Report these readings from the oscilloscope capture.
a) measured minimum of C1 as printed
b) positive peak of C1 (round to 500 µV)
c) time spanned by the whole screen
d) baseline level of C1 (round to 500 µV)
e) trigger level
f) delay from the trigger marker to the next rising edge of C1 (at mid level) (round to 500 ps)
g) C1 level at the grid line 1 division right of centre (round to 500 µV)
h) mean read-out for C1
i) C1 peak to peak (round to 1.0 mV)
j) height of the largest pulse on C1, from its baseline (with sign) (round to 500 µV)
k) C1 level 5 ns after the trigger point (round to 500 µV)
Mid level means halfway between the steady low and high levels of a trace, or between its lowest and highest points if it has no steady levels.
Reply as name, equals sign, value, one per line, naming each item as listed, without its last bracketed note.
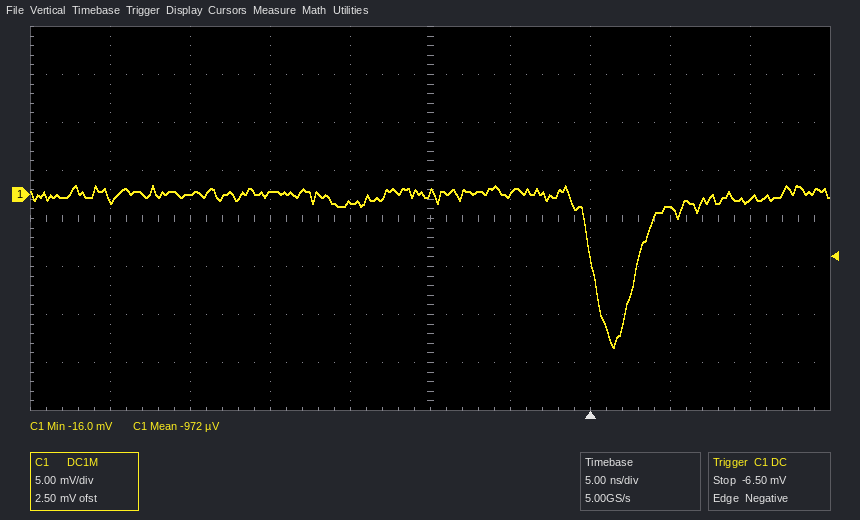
measured minimum of C1 as printed = -16.0 mV
positive peak of C1 = 1.0 mV
time spanned by the whole screen = 50 ns
baseline level of C1 = 0.0 mV
trigger level = -6.50 mV
delay from the trigger marker to the next rising edge of C1 (at mid level) = 3.0 ns
C1 level at the grid line 1 division right of centre = 0.0 mV
mean read-out for C1 = -972 µV
C1 peak to peak = 17.0 mV
height of the largest pulse on C1, from its baseline (with sign) = -16.0 mV
C1 level 5 ns after the trigger point = -1.5 mV
